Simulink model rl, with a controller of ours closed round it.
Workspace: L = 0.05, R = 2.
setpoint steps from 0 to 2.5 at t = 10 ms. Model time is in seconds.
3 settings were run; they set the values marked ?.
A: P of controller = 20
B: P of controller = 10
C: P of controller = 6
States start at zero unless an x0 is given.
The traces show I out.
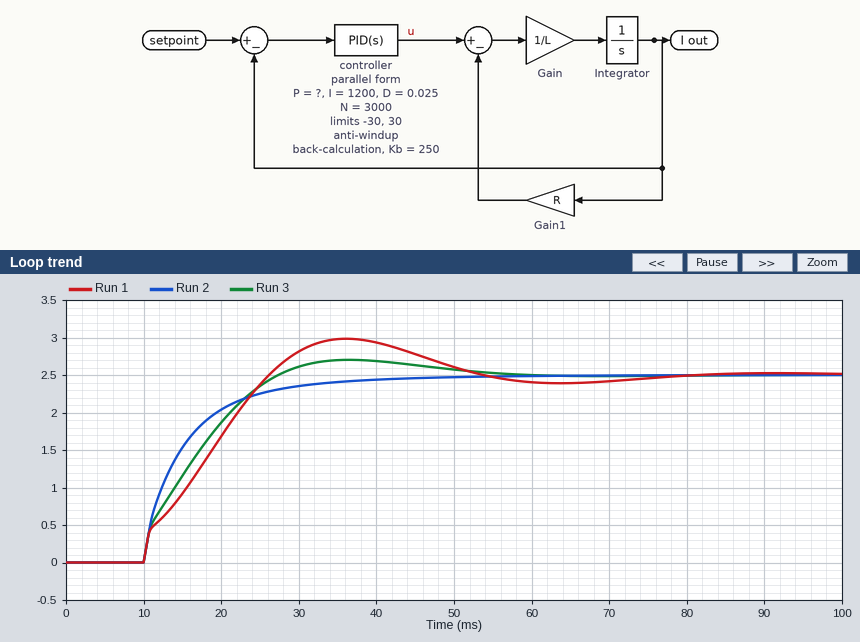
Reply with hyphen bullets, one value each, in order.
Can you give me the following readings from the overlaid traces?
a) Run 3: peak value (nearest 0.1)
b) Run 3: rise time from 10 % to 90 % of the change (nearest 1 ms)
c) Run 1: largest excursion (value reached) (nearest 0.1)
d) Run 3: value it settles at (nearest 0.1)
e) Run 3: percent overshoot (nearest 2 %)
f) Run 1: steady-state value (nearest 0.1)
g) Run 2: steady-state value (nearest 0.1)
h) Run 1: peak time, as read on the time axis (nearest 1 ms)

- 2.7
- 13 ms
- 3.0
- 2.5
- 8 %
- 2.5
- 2.5
- 36 ms
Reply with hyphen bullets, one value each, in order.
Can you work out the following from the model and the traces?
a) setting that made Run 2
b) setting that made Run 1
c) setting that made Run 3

- A
- C
- B
